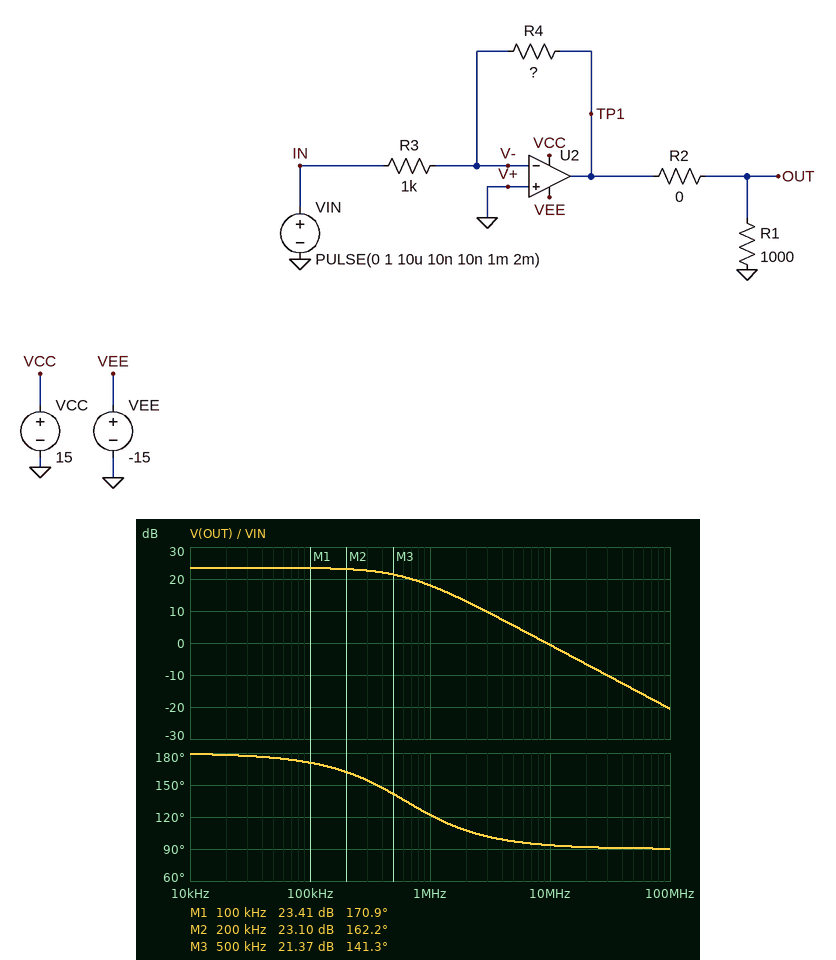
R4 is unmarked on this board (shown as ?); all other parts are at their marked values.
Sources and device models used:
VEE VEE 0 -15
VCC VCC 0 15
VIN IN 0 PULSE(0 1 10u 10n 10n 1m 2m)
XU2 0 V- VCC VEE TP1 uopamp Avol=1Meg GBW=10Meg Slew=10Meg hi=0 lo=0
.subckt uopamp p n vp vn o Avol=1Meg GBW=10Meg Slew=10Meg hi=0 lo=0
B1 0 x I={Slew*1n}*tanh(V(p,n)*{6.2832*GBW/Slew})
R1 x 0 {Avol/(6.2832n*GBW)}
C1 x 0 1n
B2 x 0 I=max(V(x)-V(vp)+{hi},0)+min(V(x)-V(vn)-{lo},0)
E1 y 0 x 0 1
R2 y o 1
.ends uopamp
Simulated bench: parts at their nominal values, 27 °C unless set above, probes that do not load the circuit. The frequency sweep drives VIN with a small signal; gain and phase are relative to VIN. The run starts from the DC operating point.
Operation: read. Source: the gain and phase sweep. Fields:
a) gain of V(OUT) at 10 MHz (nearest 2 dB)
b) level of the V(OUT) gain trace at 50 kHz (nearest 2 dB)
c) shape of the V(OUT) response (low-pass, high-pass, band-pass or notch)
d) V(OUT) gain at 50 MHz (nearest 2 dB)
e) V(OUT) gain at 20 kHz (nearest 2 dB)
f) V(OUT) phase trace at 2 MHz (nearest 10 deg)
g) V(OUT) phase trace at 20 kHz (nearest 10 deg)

0 dB
24 dB
low-pass
-14 dB
24 dB
110 deg
180 deg
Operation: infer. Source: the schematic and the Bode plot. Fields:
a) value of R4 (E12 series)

15 kΩ
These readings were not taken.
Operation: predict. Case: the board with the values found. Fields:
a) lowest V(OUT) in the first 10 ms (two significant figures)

-15 V
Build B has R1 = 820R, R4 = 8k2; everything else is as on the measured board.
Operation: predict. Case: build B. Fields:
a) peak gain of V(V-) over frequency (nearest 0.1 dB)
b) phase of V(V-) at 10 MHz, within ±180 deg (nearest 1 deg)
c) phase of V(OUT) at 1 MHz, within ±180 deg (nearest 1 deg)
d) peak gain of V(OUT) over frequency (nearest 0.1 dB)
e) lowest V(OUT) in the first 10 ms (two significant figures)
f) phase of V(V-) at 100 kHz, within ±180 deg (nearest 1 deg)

-1.0 dB
6 deg
137 deg
18.3 dB
-8.2 V
85 deg
